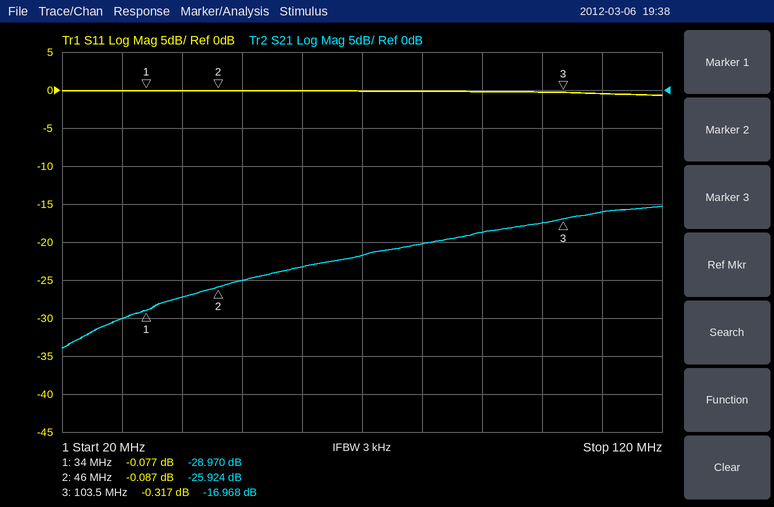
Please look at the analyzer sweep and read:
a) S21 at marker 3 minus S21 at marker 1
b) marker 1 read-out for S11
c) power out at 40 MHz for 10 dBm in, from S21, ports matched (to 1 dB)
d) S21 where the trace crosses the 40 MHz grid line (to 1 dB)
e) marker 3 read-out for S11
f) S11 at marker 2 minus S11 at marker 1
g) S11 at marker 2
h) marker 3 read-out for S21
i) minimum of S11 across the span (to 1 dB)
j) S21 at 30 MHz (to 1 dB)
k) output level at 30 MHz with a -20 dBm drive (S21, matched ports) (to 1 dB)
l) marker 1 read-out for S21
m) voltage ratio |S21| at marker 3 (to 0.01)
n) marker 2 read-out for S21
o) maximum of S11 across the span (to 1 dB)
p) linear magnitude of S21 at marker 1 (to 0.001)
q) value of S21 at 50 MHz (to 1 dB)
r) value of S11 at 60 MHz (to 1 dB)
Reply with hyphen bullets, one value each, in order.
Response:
- 12.002 dB
- -0.077 dB
- -17 dBm
- -27 dB
- -0.317 dB
- -0.010 dB
- -0.087 dB
- -16.968 dB
- -1 dB
- -30 dB
- -50 dBm
- -28.970 dB
- 0.14
- -25.924 dB
- 0 dB
- 0.036
- -25 dB
- 0 dB
